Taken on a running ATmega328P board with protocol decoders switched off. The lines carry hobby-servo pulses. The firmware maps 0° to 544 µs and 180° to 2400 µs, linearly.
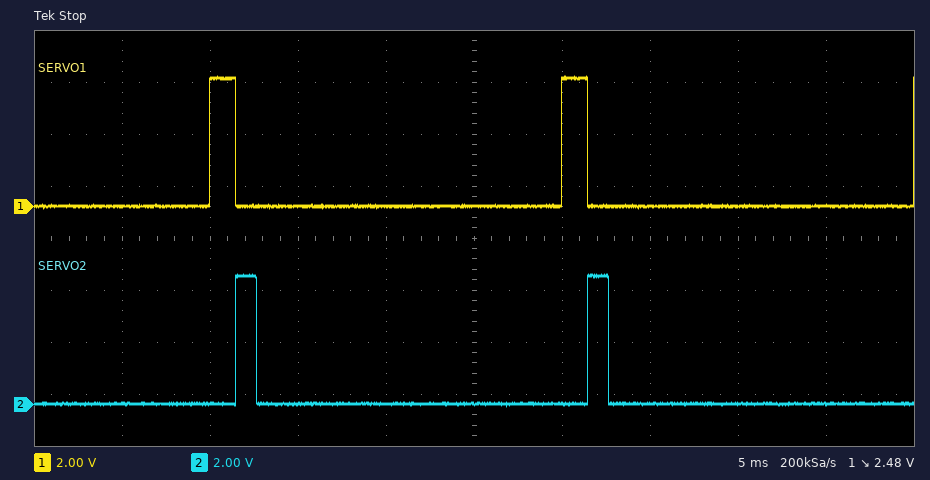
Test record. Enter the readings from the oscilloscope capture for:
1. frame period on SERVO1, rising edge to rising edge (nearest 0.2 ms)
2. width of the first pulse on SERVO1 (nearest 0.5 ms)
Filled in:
20.0 ms
1.5 ms
